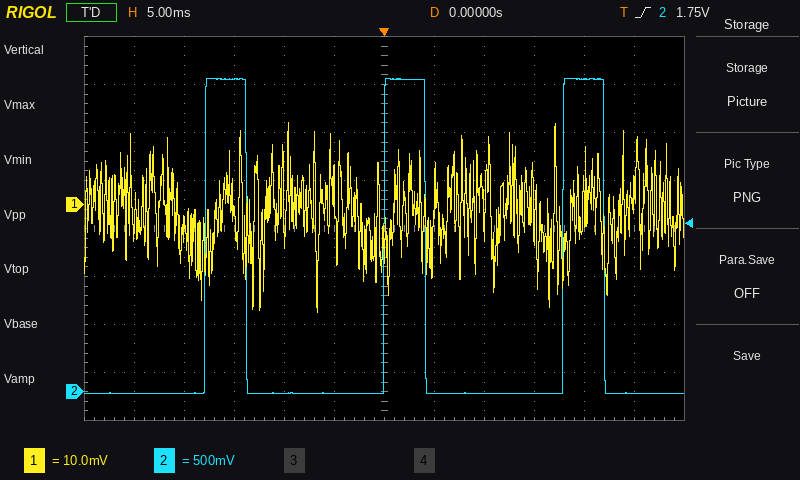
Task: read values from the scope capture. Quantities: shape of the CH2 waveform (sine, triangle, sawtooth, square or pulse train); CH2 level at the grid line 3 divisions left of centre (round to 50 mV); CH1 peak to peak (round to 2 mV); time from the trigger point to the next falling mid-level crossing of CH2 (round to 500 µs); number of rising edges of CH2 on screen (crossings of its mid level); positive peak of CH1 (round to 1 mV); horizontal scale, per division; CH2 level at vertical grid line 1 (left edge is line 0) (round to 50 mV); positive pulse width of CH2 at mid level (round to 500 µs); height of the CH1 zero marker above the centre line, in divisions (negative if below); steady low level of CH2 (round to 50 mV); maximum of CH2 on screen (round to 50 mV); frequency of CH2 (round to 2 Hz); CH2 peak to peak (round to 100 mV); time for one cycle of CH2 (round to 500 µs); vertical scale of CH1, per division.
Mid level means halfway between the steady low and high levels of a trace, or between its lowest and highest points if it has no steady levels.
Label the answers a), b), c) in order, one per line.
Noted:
a) pulse train
b) 3.25 V
c) 40 mV
d) 4.0 ms
e) 3
f) 17 mV
g) 5 ms
h) 0 mV
i) 4.0 ms
j) +0.5 div
k) 0 mV
l) 3.25 V
m) 56 Hz
n) 3.30 V
o) 18.0 ms
p) 10 mV
